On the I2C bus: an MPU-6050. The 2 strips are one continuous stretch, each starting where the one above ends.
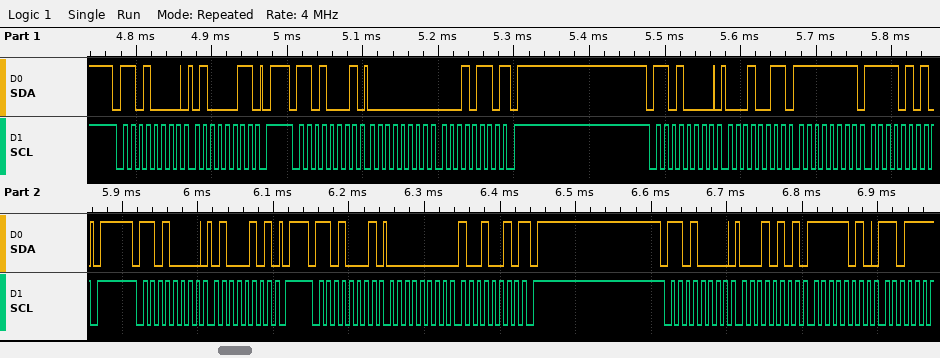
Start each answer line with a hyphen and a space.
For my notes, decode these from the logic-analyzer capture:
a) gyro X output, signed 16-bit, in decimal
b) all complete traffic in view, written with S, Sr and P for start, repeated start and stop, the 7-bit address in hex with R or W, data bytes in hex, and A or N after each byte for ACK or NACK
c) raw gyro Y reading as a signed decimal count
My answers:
- 22
- S 68W A 43 A P S 68R A 00 A 16 N P S 68W A 13 A FF A F5 A P S 68W A 45 A P S 68R A 00 A 92 N P S 68W A 15 A FA A
- 146
